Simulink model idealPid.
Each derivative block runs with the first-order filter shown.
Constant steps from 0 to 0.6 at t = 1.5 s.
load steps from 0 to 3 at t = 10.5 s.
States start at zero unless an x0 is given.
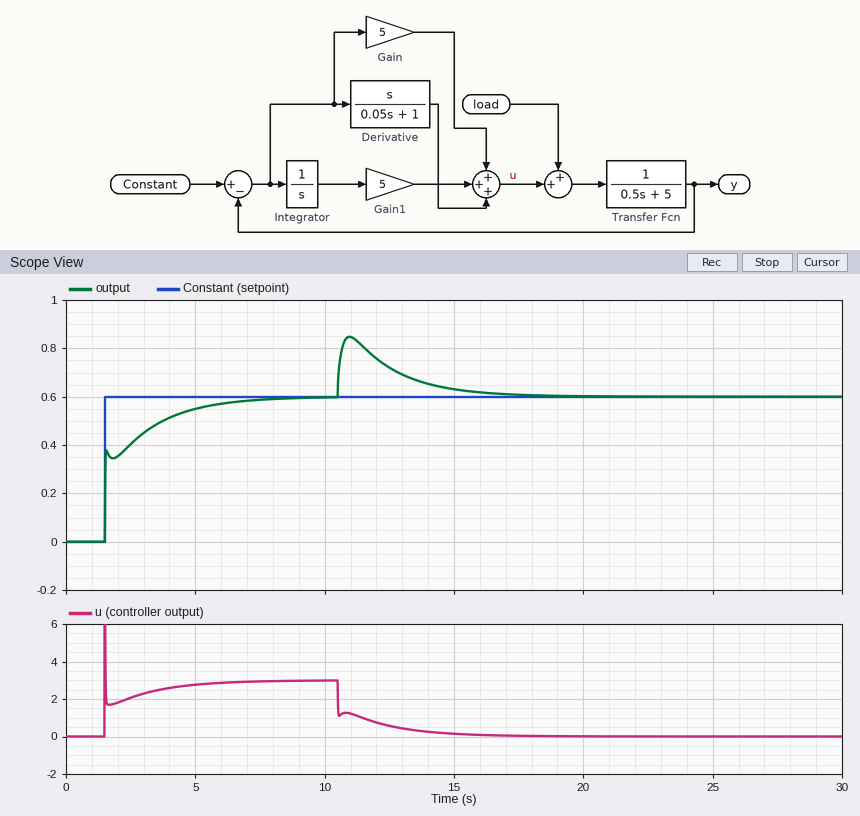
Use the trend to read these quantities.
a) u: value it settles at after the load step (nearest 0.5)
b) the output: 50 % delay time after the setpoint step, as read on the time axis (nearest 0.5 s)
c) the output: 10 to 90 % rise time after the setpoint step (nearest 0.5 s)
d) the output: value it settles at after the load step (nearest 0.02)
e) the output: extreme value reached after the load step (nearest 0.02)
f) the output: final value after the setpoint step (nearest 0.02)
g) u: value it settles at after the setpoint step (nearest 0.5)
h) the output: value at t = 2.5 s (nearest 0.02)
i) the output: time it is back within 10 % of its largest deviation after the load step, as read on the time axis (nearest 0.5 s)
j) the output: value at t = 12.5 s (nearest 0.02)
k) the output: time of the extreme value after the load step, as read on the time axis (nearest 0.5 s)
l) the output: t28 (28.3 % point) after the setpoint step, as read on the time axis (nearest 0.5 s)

0.0
1.5 s
3.0 s
0.60
0.84
0.60
3.0
0.40
15.5 s
0.72
11.0 s
1.5 s
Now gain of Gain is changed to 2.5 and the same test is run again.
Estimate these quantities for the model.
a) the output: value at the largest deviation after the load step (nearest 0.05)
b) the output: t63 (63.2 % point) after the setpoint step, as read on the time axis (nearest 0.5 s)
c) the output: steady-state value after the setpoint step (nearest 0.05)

0.90
2.5 s
0.60
